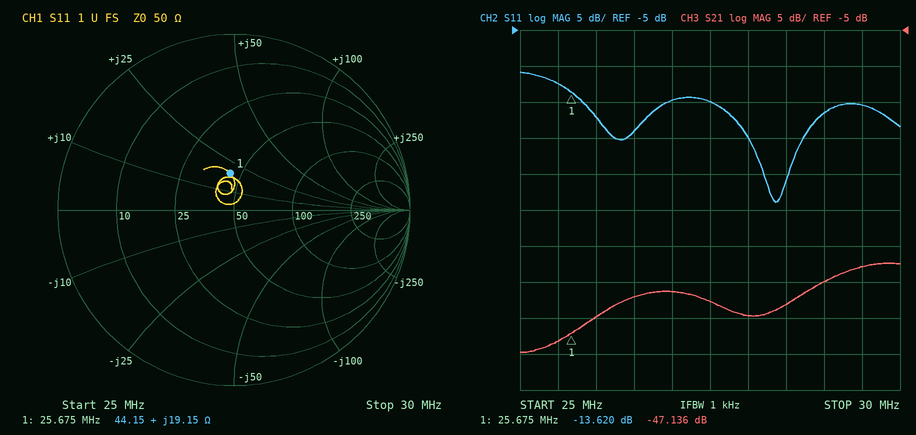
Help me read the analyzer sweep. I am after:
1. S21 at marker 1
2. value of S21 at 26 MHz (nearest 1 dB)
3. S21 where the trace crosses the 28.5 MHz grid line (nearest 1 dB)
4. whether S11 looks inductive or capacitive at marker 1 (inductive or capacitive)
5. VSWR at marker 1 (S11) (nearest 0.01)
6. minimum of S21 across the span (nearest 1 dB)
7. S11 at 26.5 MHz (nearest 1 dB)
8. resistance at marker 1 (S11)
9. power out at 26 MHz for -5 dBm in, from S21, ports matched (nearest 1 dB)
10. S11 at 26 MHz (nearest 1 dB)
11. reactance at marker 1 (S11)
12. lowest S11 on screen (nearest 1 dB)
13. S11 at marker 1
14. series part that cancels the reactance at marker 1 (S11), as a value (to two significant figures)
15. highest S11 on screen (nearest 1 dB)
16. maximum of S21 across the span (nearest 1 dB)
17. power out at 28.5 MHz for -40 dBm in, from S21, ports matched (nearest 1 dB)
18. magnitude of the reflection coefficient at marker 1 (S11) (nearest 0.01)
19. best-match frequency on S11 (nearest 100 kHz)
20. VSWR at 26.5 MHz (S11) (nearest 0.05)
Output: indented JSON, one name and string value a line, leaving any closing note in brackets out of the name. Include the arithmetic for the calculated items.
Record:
{
  "S21 at marker 1": "-47.136 dB",
  "value of S21 at 26 MHz": "-45 dB",
  "S21 where the trace crosses the 28.5 MHz grid line": "-43 dB",
  "whether S11 looks inductive or capacitive at marker 1": "inductive",
  "VSWR at marker 1 (S11)": "1.53",
  "minimum of S21 across the span": "-50 dB",
  "S11 at 26.5 MHz": "-19 dB",
  "resistance at marker 1": "44.15 Ω",
  "power out at 26 MHz for -5 dBm in, from S21, ports matched": "-5 dBm + (-45 dB) = -50 dBm",
  "S11 at 26 MHz": "-17 dB",
  "reactance at marker 1": "+19.15 Ω",
  "lowest S11 on screen": "-29 dB",
  "S11 at marker 1": "-13.620 dB",
  "series part that cancels the reactance at marker 1 (S11), as a value": "C = 1/(2π × 25.675 MHz × 19.15 Ω) ≈ 324 pF, so 320 pF to two significant figures",
  "highest S11 on screen": "-11 dB",
  "maximum of S21 across the span": "-37 dB",
  "power out at 28.5 MHz for -40 dBm in, from S21, ports matched": "-40 dBm + (-43 dB) = -83 dBm",
  "magnitude of the reflection coefficient at marker 1 (S11)": "10^(-13.62/20) ≈ 0.21",
  "best-match frequency on S11": "28.4 MHz",
  "VSWR at 26.5 MHz (S11)": "|Γ| = 10^(-19/20) = 0.1122; VSWR = (1 + 0.1122)/(1 − 0.1122) ≈ 1.25"
}
